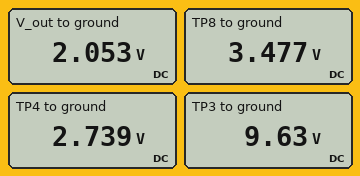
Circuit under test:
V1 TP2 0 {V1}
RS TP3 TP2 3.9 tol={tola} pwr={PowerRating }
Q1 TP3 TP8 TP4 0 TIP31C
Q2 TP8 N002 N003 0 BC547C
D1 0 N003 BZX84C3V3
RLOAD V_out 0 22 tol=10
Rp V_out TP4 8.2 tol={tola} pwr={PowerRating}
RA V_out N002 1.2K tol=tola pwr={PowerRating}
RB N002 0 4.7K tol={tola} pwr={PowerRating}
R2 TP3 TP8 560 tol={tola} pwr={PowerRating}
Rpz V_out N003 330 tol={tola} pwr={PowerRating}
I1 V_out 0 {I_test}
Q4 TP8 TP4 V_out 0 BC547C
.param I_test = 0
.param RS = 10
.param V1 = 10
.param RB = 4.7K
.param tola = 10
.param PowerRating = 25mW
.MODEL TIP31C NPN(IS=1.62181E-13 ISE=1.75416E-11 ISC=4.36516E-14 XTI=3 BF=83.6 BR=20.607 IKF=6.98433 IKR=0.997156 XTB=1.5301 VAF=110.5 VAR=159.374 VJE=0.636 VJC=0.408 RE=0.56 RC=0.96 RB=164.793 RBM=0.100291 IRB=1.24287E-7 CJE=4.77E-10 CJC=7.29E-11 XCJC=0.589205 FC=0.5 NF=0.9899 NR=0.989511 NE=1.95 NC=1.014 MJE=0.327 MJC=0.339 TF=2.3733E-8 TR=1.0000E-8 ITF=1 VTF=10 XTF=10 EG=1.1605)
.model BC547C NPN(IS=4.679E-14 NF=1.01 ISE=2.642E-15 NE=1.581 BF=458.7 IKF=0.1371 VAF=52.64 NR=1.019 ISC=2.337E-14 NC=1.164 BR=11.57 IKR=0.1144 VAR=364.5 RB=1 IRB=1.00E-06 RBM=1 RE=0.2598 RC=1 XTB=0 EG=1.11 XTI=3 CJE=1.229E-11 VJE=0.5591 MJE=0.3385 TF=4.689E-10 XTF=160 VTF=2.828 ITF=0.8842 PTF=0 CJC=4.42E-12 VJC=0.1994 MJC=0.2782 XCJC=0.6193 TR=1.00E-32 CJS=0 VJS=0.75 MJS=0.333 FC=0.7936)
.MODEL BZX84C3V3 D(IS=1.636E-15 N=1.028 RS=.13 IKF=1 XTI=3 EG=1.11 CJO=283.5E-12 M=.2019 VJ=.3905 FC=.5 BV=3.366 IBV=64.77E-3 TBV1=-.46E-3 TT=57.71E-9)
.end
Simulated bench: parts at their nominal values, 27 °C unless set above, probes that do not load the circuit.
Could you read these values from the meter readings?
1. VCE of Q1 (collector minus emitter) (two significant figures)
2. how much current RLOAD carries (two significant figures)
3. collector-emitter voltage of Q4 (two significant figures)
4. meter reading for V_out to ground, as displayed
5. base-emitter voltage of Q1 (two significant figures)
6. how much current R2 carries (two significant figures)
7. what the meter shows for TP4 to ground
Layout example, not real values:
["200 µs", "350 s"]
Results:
["6.9 V", "93 mA", "1.4 V", "2.053 V", "740 mV", "11 mA", "2.739 V"]
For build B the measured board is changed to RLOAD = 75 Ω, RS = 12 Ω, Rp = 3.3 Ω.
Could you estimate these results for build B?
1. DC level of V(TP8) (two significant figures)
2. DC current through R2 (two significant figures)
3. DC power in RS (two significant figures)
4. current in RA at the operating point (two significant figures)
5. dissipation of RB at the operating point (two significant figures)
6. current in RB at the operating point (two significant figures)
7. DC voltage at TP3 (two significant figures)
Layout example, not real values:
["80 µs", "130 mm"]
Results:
["6.0 V", "5.5 mA", "72 mW", "860 µA", "3.4 mW", "850 µA", "9.1 V"]
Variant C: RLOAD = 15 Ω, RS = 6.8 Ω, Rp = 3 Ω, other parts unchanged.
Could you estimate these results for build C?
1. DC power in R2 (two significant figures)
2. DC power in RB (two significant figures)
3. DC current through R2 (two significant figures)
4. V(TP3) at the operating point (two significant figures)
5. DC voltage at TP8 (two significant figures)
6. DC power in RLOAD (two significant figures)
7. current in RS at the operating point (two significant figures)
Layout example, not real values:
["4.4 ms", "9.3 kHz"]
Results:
["24 mW", "1.5 mW", "6.5 mA", "8.5 V", "4.8 V", "740 mW", "220 mA"]
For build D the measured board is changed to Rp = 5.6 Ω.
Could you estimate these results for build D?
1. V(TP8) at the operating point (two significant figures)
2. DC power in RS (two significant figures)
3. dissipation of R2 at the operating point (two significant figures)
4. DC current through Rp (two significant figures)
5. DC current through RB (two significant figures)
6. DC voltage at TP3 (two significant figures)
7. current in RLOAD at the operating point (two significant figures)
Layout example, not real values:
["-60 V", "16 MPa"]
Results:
["4.3 V", "65 mW", "49 mW", "120 mA", "480 µA", "9.5 V", "130 mA"]
